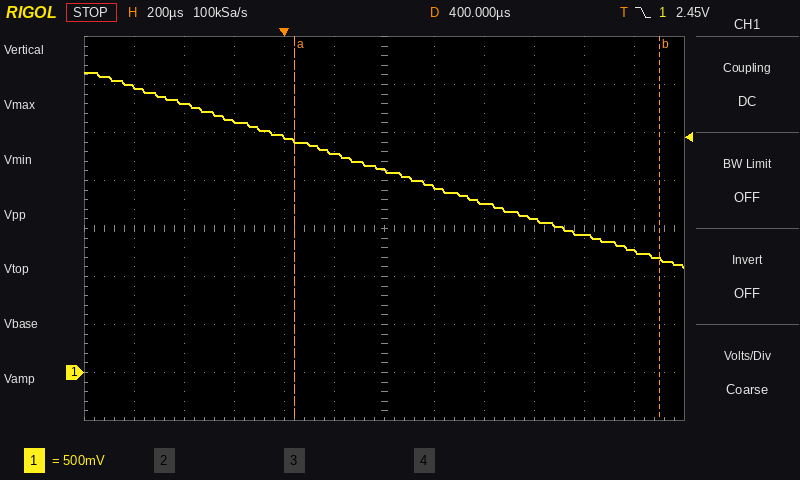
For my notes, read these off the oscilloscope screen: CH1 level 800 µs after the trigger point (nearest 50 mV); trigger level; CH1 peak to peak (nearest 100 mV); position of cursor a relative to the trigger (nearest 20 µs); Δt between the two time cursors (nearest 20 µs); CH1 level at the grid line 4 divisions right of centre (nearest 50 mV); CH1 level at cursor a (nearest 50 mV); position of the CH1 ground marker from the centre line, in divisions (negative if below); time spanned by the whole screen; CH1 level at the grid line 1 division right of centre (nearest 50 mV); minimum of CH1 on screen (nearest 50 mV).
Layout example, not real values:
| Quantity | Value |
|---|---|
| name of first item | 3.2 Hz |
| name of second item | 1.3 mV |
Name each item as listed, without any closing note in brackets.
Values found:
| Quantity | Value |
|---|---|
| CH1 level 800 µs after the trigger point | 1.75 V |
| trigger level | 2.45 V |
| CH1 peak to peak | 2.00 V |
| position of cursor a relative to the trigger | +40 µs |
| Δt between the two time cursors | 1.46 ms |
| CH1 level at the grid line 4 divisions right of centre | 1.45 V |
| CH1 level at cursor a | 2.40 V |
| position of the CH1 ground marker from the centre line, in divisions | -3.0 div |
| time spanned by the whole screen | 2.4 ms |
| CH1 level at the grid line 1 division right of centre | 1.95 V |
| minimum of CH1 on screen | 1.10 V |
